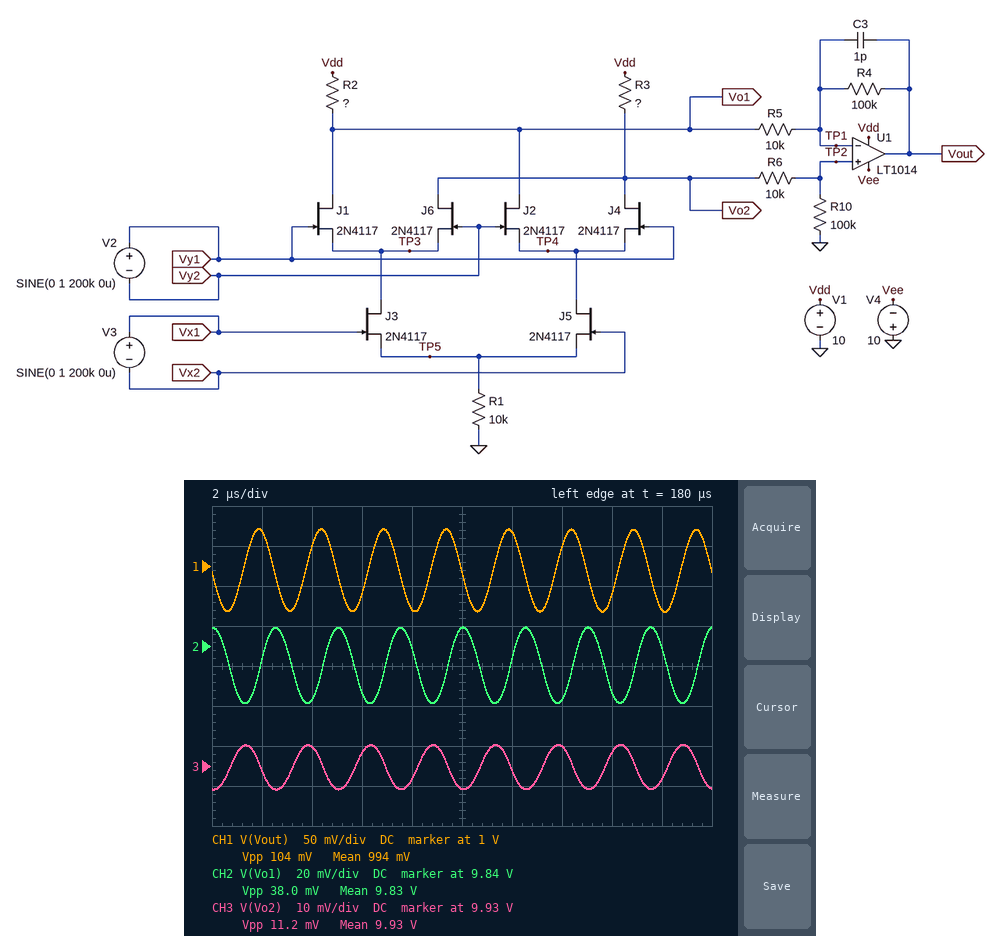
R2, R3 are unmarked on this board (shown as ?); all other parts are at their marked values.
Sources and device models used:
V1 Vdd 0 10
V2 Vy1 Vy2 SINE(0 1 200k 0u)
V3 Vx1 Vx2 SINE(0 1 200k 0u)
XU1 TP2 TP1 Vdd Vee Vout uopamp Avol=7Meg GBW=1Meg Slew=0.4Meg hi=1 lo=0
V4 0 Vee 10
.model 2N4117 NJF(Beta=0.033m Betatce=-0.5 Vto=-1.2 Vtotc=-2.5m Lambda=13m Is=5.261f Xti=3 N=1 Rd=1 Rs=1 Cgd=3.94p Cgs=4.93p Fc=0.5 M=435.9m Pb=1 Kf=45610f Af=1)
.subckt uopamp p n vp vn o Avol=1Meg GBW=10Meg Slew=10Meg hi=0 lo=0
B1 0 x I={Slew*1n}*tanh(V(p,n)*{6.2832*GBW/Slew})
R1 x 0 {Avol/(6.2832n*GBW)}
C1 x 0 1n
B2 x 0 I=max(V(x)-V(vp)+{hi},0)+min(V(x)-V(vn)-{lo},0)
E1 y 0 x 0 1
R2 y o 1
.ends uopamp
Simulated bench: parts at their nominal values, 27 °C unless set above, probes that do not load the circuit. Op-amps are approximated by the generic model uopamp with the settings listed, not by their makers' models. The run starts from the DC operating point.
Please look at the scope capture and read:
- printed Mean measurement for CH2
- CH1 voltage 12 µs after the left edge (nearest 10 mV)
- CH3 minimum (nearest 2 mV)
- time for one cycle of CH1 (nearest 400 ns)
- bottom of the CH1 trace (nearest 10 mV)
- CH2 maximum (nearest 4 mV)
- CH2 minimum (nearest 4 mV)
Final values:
9.83 V
1.04 V
9.924 V
2.4 µs
940 mV
9.848 V
9.812 V
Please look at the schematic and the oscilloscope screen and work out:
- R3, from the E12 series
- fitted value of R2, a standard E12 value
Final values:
560 Ω
1.2 kΩ
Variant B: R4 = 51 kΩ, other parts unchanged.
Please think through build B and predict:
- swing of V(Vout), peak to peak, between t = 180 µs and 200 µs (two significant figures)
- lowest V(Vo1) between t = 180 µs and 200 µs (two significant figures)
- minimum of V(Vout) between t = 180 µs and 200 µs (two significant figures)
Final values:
92 mV
9.8 V
4.9 V
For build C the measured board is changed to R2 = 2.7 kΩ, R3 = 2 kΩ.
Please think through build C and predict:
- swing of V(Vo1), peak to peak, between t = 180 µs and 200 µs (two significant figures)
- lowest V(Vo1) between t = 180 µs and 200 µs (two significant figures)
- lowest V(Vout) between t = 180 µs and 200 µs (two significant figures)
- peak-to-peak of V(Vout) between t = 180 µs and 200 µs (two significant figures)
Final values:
84 mV
9.6 V
1.1 V
230 mV
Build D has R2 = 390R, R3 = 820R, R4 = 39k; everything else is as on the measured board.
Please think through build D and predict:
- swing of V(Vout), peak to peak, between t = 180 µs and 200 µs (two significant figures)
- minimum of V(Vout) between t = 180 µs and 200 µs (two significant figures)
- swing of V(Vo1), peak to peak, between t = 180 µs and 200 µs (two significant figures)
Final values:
54 mV
5.3 V
12 mV
